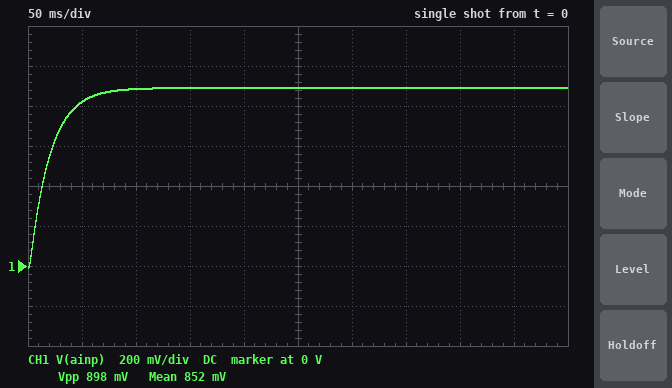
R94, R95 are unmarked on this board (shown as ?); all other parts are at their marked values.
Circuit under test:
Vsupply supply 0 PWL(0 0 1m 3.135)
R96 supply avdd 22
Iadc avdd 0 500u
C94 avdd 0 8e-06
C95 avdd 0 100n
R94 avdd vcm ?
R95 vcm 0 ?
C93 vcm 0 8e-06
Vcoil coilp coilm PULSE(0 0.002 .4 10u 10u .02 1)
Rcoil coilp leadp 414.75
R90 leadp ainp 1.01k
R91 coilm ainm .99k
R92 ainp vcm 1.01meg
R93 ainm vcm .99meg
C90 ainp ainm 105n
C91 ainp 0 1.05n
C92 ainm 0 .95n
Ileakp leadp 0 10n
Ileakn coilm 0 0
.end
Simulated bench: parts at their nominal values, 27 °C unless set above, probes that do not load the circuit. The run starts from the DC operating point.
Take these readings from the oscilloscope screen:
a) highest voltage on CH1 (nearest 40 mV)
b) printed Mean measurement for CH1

880 mV
852 mV
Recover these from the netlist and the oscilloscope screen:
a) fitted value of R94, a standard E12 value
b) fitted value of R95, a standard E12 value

8.2 kΩ
3.3 kΩ
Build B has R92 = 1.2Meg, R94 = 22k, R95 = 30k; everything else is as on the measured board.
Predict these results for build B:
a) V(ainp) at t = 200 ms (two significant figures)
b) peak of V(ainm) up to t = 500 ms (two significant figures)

1.5 V
1.8 V
